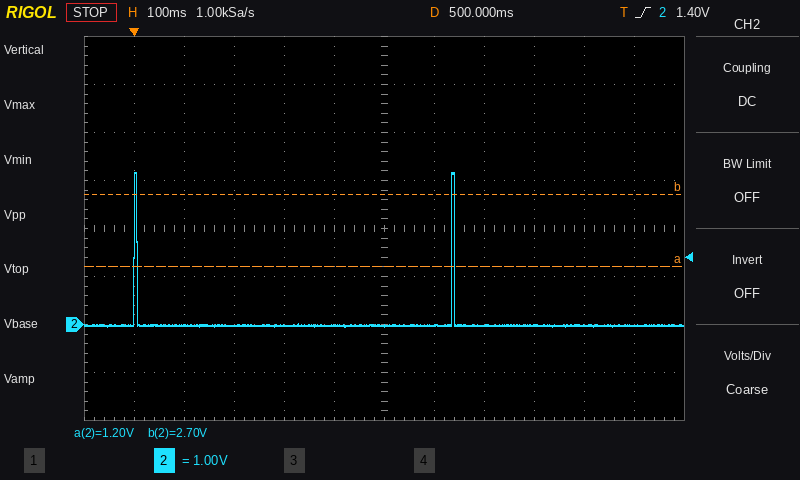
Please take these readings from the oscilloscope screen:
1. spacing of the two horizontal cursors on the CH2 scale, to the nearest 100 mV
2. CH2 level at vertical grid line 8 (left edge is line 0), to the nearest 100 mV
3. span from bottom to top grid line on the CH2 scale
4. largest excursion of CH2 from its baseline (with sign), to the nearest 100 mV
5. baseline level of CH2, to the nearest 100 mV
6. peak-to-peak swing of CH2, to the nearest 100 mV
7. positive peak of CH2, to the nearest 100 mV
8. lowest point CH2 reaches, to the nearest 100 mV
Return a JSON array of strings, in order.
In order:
["1.5 V", "0.0 V", "8 V", "+3.2 V", "0.0 V", "3.2 V", "3.2 V", "0.0 V"]
